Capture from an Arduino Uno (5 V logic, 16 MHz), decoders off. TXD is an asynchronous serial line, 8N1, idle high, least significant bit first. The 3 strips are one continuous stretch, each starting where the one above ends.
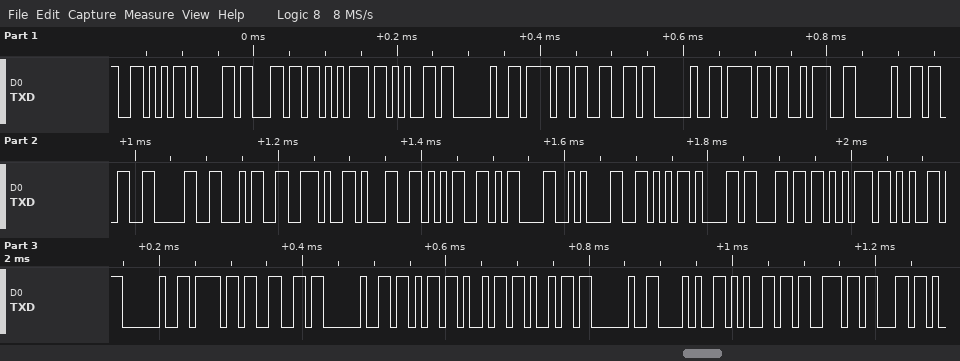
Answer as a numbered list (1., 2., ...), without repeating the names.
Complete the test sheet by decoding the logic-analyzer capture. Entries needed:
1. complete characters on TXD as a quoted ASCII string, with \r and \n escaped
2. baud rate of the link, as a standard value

1. "Value of o: 304.15\r\nValue of kii (esc"
2. 115200 baud
